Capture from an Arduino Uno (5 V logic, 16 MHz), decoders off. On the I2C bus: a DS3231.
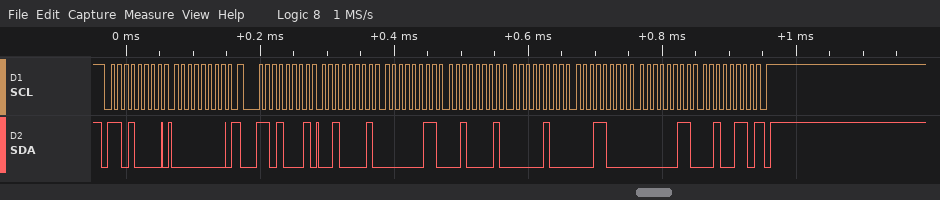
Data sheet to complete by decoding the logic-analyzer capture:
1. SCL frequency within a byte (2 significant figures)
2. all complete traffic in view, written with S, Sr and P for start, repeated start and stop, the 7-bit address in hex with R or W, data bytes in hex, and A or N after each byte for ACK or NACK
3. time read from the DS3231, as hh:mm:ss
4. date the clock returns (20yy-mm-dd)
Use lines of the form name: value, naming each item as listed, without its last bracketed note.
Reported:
SCL frequency within a byte: 100 kHz
all complete traffic in view, written with S, Sr and P for start, repeated start and stop, the 7-bit address in hex with R or W, data bytes in hex, and A or N after each byte for ACK or NACK: S 68W A 00 A Sr 68R A 21 A 03 A 21 A 04 A 18 A 03 A 26 N P
time read from the DS3231, as hh:mm:ss: 21:03:21
date the clock returns: 2026-03-18
